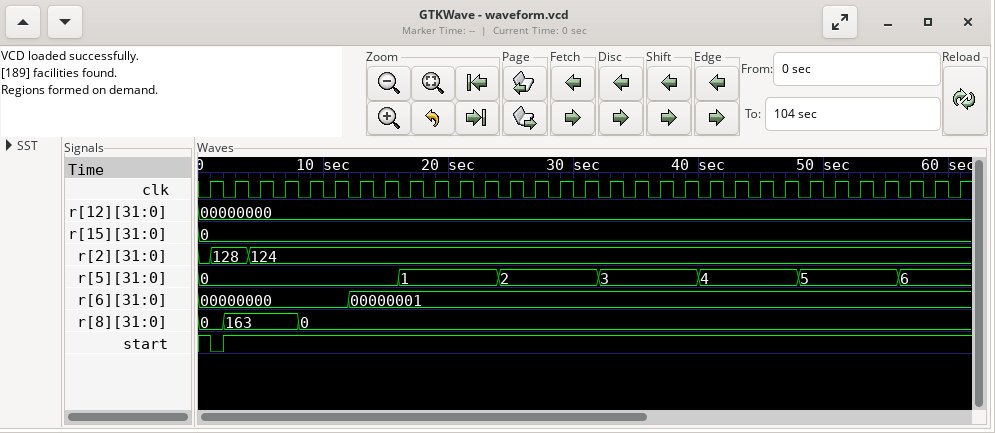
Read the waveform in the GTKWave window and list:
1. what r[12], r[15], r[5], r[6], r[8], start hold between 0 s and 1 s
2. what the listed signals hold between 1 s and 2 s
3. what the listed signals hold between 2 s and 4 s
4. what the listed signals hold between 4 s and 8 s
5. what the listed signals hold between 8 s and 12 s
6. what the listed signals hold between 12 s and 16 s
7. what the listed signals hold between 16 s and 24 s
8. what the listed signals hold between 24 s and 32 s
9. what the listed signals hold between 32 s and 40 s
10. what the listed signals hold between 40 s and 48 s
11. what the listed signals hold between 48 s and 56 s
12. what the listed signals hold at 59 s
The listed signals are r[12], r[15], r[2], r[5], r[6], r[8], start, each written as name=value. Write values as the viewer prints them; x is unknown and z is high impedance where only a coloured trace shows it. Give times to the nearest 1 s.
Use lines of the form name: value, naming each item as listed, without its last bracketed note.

what r[12], r[15], r[5], r[6], r[8], start hold between 0 s and 1 s: r[12]=00000000, r[15]=0, r[5]=0, r[6]=00000000, r[8]=0, start=1
what the listed signals hold between 1 s and 2 s: r[12]=00000000, r[15]=0, r[2]=128, r[5]=0, r[6]=00000000, r[8]=0, start=0
what the listed signals hold between 2 s and 4 s: r[12]=00000000, r[15]=0, r[2]=128, r[5]=0, r[6]=00000000, r[8]=163, start=1
what the listed signals hold between 4 s and 8 s: r[12]=00000000, r[15]=0, r[2]=124, r[5]=0, r[6]=00000000, r[8]=163, start=1
what the listed signals hold between 8 s and 12 s: r[12]=00000000, r[15]=0, r[2]=124, r[5]=0, r[6]=00000000, r[8]=0, start=1
what the listed signals hold between 12 s and 16 s: r[12]=00000000, r[15]=0, r[2]=124, r[5]=0, r[6]=00000001, r[8]=0, start=1
what the listed signals hold between 16 s and 24 s: r[12]=00000000, r[15]=0, r[2]=124, r[5]=1, r[6]=00000001, r[8]=0, start=1
what the listed signals hold between 24 s and 32 s: r[12]=00000000, r[15]=0, r[2]=124, r[5]=2, r[6]=00000001, r[8]=0, start=1
what the listed signals hold between 32 s and 40 s: r[12]=00000000, r[15]=0, r[2]=124, r[5]=3, r[6]=00000001, r[8]=0, start=1
what the listed signals hold between 40 s and 48 s: r[12]=00000000, r[15]=0, r[2]=124, r[5]=4, r[6]=00000001, r[8]=0, start=1
what the listed signals hold between 48 s and 56 s: r[12]=00000000, r[15]=0, r[2]=124, r[5]=5, r[6]=00000001, r[8]=0, start=1
what the listed signals hold at 59 s: r[12]=00000000, r[15]=0, r[2]=124, r[5]=6, r[6]=00000001, r[8]=0, start=1
